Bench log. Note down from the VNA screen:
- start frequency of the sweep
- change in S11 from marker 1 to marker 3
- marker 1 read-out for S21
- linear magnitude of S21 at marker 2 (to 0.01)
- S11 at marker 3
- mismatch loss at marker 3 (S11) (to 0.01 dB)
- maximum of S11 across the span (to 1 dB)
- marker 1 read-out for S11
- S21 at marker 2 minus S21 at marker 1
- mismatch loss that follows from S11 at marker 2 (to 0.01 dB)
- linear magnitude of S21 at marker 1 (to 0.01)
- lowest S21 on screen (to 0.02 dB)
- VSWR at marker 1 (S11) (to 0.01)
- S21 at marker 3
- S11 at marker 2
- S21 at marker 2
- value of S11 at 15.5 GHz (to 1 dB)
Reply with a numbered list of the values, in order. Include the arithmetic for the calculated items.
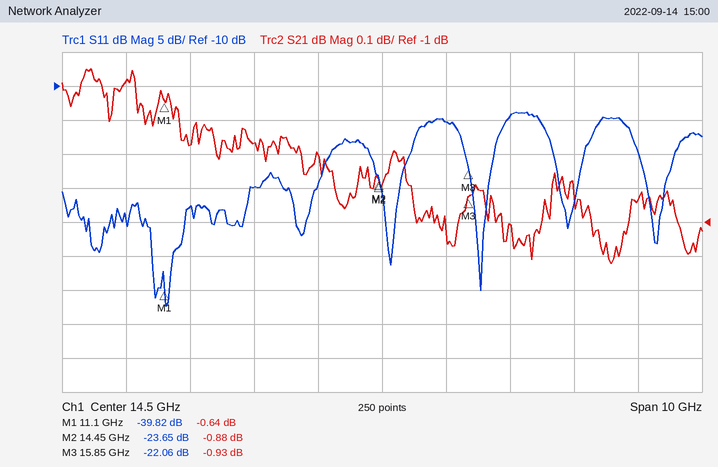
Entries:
1. 9.5 GHz
2. -22.06 − (-39.82) = 17.76 dB
3. -0.64 dB
4. 10^(-0.88/20) ≈ 0.90
5. -22.06 dB
6. −10 log10(1 − 10^(-22.06/10)) ≈ 0.03 dB
7. -14 dB
8. -39.82 dB
9. -0.88 − (-0.64) = -0.24 dB
10. −10 log10(1 − 10^(-23.65/10)) ≈ 0.02 dB
11. 10^(-0.64/20) ≈ 0.93
12. -1.12 dB
13. (1 + 0.0102)/(1 − 0.0102) ≈ 1.02
14. -0.93 dB
15. -23.65 dB
16. -0.88 dB
17. -15 dB
